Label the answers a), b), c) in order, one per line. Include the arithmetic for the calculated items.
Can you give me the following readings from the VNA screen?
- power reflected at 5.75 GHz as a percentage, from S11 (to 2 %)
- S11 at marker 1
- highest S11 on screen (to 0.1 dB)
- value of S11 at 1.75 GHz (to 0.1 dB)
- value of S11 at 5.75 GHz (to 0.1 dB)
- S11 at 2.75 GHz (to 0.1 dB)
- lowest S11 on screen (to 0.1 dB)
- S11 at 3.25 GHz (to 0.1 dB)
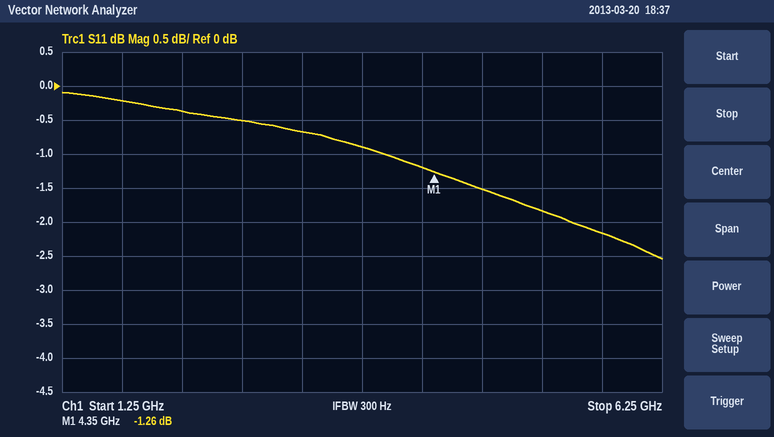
a) 10^(-2.2/10) ≈ 60 %
b) -1.26 dB
c) -0.1 dB
d) -0.2 dB
e) -2.2 dB
f) -0.5 dB
g) -2.5 dB
h) -0.7 dB
